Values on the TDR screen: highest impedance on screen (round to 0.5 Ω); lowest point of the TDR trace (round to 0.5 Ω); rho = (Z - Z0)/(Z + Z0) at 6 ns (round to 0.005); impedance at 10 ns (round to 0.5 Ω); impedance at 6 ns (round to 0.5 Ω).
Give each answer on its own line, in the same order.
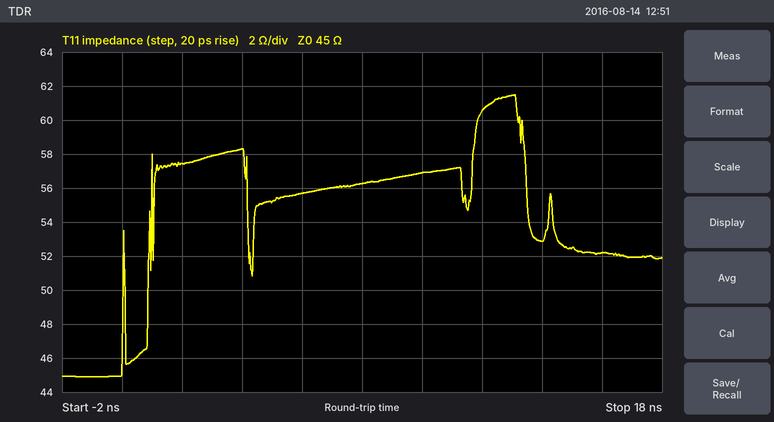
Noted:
61.5 Ω
45.0 Ω
+0.105
57.0 Ω
55.5 Ω
